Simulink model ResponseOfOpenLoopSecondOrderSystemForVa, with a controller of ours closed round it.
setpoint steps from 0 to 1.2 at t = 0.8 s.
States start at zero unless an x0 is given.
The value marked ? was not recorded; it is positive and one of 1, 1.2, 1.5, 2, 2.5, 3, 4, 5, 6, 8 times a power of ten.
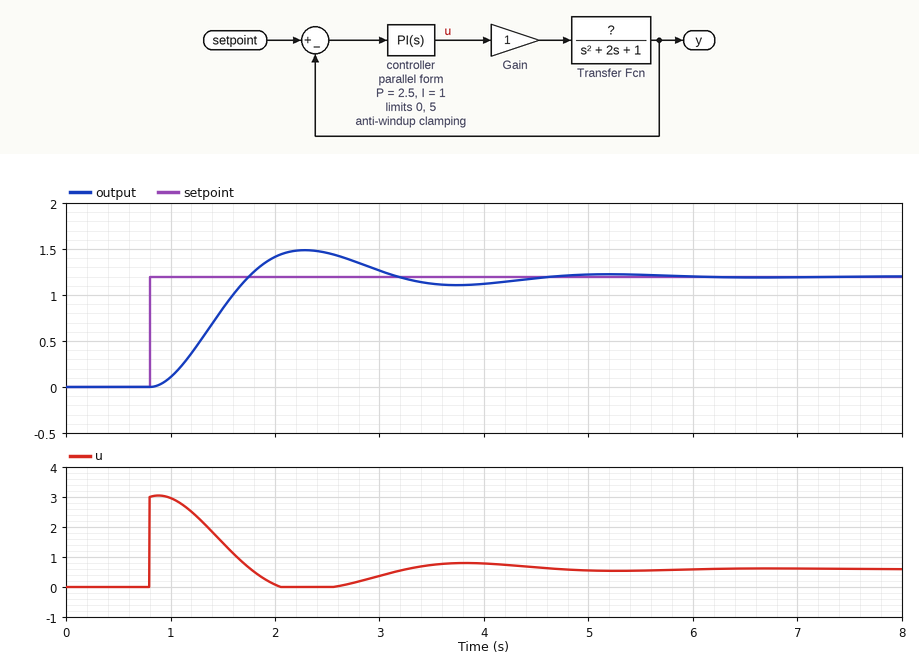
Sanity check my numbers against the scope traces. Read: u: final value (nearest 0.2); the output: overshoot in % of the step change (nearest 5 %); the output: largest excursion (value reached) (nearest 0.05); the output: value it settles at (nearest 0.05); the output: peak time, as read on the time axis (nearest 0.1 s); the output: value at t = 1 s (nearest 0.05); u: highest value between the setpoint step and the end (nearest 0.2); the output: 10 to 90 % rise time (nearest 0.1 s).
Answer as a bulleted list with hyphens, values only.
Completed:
- 0.6
- 25 %
- 1.50
- 1.20
- 2.3 s
- 0.10
- 3.0
- 0.6 s
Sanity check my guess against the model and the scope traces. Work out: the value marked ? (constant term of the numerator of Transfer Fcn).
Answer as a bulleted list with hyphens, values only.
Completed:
- 2
